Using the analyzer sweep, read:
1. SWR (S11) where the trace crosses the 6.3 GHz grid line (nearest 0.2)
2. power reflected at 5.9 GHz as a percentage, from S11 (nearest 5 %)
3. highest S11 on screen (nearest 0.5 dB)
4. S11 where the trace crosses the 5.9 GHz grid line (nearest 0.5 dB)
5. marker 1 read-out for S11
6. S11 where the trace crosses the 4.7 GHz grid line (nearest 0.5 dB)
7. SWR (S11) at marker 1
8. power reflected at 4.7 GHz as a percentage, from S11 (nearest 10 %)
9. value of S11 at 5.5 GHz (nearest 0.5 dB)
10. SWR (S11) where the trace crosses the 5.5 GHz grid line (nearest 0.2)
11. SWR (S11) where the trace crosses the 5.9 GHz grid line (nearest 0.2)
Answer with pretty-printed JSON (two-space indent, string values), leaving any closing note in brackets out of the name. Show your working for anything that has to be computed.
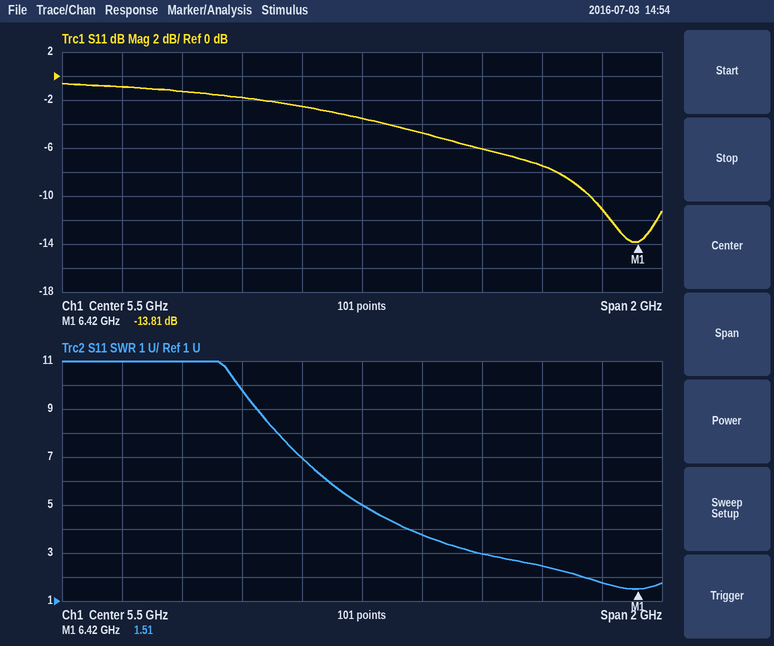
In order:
{
  "SWR (S11) where the trace crosses the 6.3 GHz grid line": "1.8",
  "power reflected at 5.9 GHz as a percentage, from S11": "10^(-6/10) ≈ 25 %",
  "highest S11 on screen": "-0.5 dB",
  "S11 where the trace crosses the 5.9 GHz grid line": "-6.0 dB",
  "marker 1 read-out for S11": "-13.81 dB",
  "S11 where the trace crosses the 4.7 GHz grid line": "-1.0 dB",
  "SWR (S11) at marker 1": "1.51",
  "power reflected at 4.7 GHz as a percentage, from S11": "10^(-1/10) ≈ 79.4 %, so 80 % to the nearest 10 %",
  "value of S11 at 5.5 GHz": "-3.5 dB",
  "SWR (S11) where the trace crosses the 5.5 GHz grid line": "5.0",
  "SWR (S11) where the trace crosses the 5.9 GHz grid line": "3.0"
}
